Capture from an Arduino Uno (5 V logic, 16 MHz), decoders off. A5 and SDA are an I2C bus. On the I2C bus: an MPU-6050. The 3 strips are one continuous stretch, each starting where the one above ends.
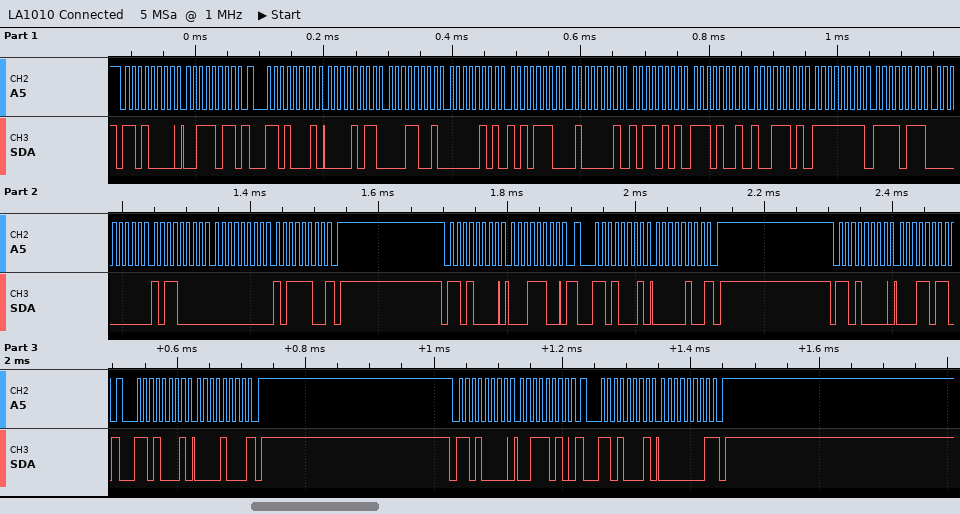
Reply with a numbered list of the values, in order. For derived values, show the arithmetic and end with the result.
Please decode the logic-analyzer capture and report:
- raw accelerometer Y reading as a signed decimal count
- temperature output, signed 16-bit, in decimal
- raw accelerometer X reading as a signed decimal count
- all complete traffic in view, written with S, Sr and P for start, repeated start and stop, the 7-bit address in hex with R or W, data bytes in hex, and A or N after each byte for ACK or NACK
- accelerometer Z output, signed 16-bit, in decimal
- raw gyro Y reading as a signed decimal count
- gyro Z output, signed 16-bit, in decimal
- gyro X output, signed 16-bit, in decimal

1. 0x05AE = 1454
2. 0xE99D = -5731
3. 0x0B19 = 2841
4. S 68W A 3B A Sr 68R A 0B A 19 A 05 A AE A 41 A B5 A E9 A 9D A FF A F7 A 00 A B0 A 00 A BC N P S 68W A 1C A Sr 68R A 04 N P S 68W A 1B A Sr 68R A 08 N P S 68W A 3A A Sr 68R A 01 N P
5. 0x41B5 = 16821
6. 0x00B0 = 176
7. 0x00BC = 188
8. 0xFFF7 = -9
